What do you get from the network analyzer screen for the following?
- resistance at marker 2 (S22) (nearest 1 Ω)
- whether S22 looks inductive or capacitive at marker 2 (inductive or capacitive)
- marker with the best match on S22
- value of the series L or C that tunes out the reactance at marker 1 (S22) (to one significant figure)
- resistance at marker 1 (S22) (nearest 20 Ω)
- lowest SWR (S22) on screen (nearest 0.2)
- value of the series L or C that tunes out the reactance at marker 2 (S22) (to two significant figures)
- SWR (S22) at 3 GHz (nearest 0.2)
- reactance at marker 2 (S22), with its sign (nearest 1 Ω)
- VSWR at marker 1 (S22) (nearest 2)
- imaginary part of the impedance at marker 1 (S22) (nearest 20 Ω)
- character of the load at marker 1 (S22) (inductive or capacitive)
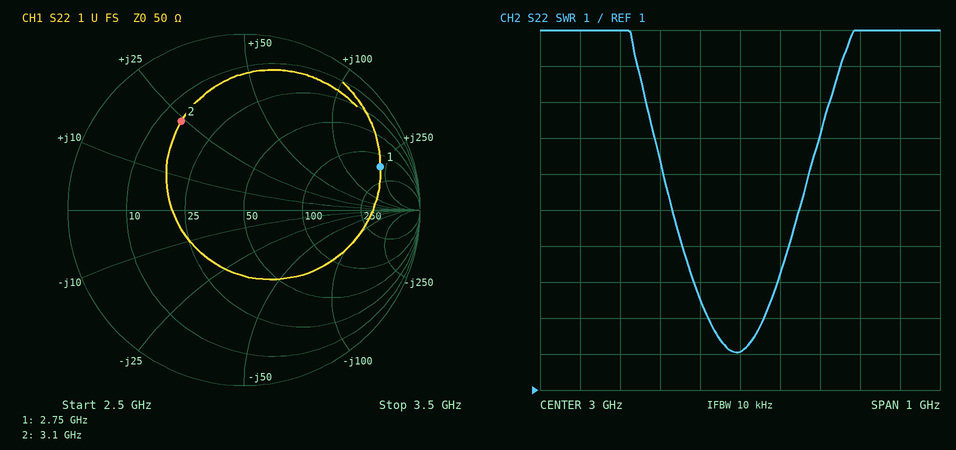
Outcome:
15 Ω
inductive
marker 2
300 fF
160 Ω
2.0
2.1 pF
2.0
+24 Ω
10
+220 Ω
inductive
